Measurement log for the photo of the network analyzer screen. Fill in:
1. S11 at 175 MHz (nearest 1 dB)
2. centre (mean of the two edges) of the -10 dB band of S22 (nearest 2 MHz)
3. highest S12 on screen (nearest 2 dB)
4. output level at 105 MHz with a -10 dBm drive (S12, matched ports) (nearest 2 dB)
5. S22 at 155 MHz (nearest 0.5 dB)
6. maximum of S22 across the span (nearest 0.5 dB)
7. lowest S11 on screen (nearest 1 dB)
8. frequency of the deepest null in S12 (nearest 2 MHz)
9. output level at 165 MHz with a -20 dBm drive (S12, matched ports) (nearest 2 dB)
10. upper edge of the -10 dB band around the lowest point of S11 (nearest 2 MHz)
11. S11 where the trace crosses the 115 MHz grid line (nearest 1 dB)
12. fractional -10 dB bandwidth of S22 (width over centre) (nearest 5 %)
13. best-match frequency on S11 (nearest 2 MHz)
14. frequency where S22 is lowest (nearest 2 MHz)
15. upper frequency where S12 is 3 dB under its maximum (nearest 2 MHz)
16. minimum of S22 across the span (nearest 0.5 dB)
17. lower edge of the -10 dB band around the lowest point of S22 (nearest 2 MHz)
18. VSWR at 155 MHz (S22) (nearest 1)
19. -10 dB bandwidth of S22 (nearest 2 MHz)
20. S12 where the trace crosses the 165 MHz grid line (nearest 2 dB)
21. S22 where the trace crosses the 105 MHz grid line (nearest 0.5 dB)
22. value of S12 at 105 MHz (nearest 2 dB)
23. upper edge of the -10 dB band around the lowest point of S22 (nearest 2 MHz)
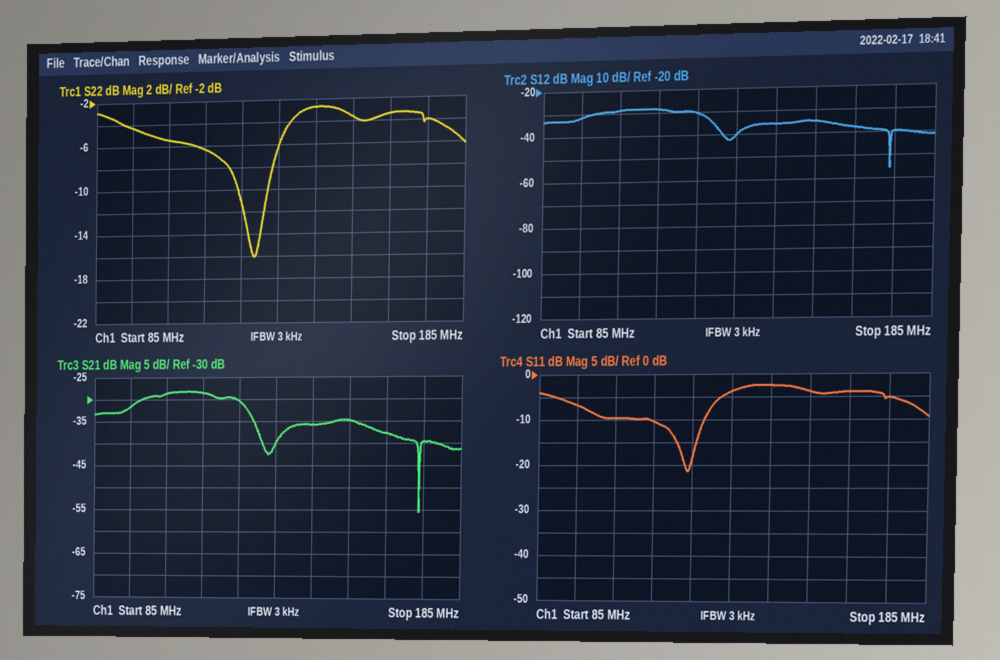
-5 dB
128 MHz
-28 dB
-38 dBm
-3.5 dB
-2.5 dB
-21 dB
174 MHz
-58 dBm
128 MHz
-10 dB
5 %
124 MHz
128 MHz
126 MHz
-16.0 dB
124 MHz
5
8 MHz
-38 dB
-5.5 dB
-28 dB
132 MHz
